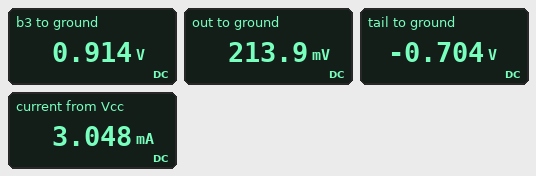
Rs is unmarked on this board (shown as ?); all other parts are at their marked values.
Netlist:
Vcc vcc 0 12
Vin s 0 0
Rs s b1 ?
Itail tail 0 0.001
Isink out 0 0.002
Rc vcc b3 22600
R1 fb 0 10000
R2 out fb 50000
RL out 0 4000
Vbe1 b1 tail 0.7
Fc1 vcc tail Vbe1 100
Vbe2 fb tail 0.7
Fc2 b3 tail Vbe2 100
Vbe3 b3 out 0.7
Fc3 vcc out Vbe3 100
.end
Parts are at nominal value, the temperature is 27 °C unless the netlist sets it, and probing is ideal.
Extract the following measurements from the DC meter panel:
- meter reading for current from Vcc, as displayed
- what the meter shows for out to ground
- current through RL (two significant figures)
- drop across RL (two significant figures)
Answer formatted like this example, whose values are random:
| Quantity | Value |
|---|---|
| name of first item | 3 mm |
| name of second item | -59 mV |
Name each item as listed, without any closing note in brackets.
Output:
| Quantity | Value |
|---|---|
| meter reading for current from Vcc, as displayed | 3.048 mA |
| what the meter shows for out to ground | 213.9 mV |
| current through RL | 53 µA |
| drop across RL | 210 mV |
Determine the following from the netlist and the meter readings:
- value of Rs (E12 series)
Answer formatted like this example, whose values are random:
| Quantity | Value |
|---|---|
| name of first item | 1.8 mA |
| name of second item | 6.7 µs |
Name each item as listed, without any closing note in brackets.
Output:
| Quantity | Value |
|---|---|
| value of Rs | 680 Ω |
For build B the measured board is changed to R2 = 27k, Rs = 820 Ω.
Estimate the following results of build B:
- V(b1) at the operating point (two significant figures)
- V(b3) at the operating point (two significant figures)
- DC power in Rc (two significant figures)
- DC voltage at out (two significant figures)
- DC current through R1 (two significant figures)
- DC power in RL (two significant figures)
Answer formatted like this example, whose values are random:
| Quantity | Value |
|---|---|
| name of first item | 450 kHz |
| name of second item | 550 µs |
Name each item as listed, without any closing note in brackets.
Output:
| Quantity | Value |
|---|---|
| V(b1) at the operating point | -4.2 mV |
| V(b3) at the operating point | 810 mV |
| DC power in Rc | 5.5 mW |
| DC voltage at out | 110 mV |
| DC current through R1 | 420 nA |
| DC power in RL | 3.2 µW |
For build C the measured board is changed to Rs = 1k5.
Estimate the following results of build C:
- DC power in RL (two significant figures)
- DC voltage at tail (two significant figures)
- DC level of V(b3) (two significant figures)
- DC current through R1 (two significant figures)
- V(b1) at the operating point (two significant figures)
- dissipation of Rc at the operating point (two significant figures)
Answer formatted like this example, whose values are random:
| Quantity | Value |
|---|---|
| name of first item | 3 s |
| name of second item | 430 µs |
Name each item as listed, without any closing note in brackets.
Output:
| Quantity | Value |
|---|---|
| DC power in RL | 8.9 µW |
| DC voltage at tail | -710 mV |
| DC level of V(b3) | 890 mV |
| DC current through R1 | 780 nA |
| V(b1) at the operating point | -7.8 mV |
| dissipation of Rc at the operating point | 5.5 mW |
